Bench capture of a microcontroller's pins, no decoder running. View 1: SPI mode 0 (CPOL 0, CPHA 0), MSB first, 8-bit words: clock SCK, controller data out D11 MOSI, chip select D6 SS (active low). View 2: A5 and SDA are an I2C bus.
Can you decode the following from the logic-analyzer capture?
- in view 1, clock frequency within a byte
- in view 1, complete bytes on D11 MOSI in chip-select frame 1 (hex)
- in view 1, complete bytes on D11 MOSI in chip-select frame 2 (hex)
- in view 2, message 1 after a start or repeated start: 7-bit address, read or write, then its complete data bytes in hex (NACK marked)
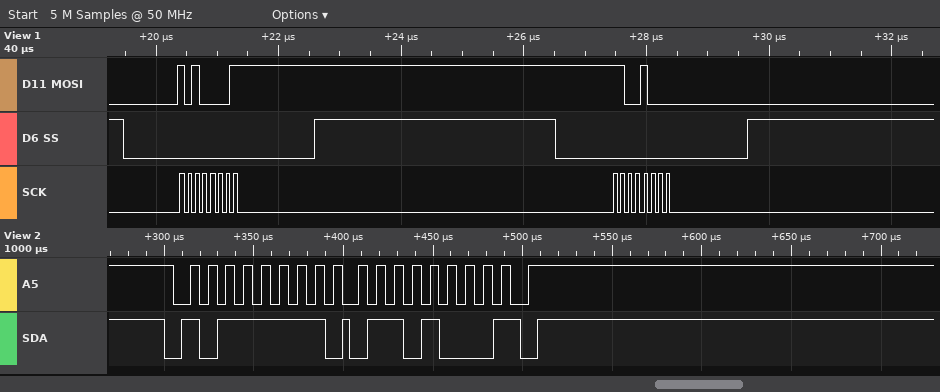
8 MHz
0xA1
0xC8
0x5F read: 68 NACK
